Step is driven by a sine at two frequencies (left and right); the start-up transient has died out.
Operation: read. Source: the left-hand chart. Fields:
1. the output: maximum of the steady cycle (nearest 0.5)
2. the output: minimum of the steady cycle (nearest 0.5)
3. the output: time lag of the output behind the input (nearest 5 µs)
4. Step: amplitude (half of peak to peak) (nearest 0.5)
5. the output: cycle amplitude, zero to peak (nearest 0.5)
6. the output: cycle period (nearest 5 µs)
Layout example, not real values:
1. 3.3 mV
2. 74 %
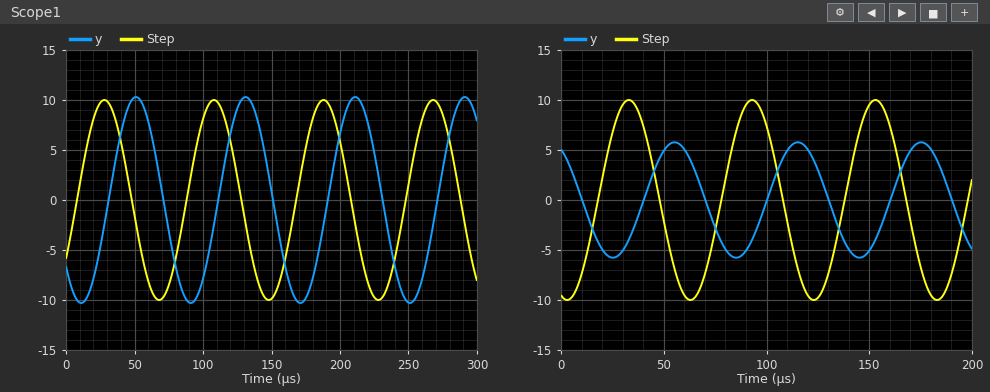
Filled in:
1. 10.5
2. -10.5
3. 25 µs
4. 10.0
5. 10.5
6. 80 µs
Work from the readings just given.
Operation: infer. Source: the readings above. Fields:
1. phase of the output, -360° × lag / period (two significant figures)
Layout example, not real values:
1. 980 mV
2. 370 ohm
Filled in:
1. -110°
